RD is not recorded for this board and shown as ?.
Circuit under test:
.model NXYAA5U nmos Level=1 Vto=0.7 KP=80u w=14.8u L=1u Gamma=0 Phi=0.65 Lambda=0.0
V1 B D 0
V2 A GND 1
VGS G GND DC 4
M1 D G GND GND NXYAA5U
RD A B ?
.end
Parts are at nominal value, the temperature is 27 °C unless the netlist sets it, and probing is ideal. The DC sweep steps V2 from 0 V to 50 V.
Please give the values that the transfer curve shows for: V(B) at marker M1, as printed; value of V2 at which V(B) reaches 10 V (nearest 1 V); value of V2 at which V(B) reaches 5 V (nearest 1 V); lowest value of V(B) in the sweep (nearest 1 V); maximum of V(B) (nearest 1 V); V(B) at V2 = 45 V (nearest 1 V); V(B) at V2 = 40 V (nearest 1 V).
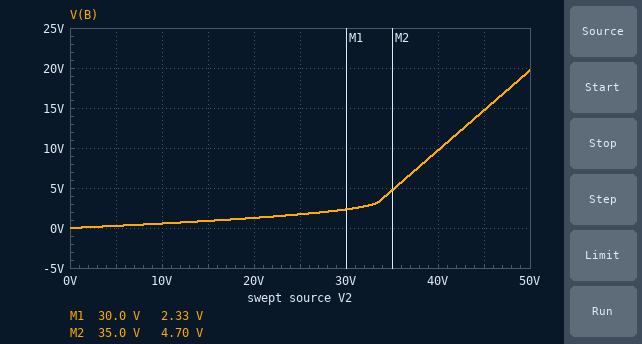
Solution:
2.33 V
40 V
35 V
0 V
20 V
15 V
10 V
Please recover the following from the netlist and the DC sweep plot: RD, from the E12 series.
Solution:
4.7 kΩ
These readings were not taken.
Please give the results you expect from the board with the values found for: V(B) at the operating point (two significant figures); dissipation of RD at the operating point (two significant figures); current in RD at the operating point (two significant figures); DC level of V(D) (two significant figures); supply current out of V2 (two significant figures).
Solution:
52 mV
190 µW
200 µA
52 mV
200 µA
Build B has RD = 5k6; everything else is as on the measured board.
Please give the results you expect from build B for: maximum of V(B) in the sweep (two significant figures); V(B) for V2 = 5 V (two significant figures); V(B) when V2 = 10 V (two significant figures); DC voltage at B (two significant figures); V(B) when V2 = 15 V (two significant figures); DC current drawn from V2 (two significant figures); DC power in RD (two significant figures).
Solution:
14 V
230 mV
470 mV
44 mV
730 mV
170 µA
160 µW
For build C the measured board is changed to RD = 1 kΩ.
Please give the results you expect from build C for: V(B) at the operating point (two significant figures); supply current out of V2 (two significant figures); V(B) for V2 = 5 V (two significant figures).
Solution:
210 mV
790 µA
1.2 V
